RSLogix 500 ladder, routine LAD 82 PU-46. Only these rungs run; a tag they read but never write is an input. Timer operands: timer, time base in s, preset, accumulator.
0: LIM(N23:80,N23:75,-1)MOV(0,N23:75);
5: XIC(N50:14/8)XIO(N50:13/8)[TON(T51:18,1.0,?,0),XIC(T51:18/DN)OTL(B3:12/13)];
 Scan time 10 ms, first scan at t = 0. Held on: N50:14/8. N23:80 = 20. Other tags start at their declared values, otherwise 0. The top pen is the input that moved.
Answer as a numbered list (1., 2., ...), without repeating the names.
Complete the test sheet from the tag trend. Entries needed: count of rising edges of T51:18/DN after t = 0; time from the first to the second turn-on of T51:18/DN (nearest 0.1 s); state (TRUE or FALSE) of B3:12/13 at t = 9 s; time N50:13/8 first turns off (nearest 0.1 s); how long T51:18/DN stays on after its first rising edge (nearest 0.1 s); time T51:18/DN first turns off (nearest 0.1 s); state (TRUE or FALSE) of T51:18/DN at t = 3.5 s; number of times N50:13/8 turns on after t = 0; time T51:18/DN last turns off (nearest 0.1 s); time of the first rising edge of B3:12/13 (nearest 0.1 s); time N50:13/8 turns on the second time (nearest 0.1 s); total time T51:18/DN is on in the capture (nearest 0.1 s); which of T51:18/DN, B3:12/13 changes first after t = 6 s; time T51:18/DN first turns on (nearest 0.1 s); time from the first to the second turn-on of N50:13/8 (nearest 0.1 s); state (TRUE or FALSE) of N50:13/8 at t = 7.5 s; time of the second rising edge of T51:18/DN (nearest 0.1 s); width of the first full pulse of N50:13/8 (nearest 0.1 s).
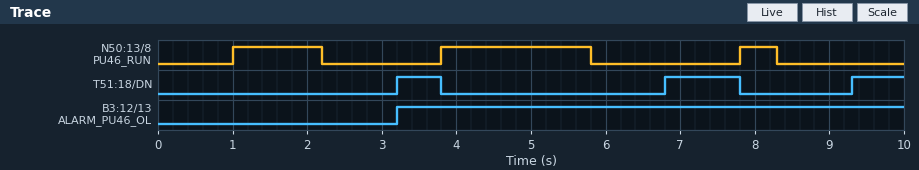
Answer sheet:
1. 3
2. 3.6 s
3. TRUE
4. 2.2 s
5. 0.6 s
6. 3.8 s
7. TRUE
8. 3
9. 7.8 s
10. 3.2 s
11. 3.8 s
12. 2.3 s
13. T51:18/DN
14. 3.2 s
15. 2.8 s
16. FALSE
17. 6.8 s
18. 1.2 s
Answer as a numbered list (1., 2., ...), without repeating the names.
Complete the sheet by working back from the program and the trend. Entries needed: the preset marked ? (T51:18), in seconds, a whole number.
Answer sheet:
1. 1 s
